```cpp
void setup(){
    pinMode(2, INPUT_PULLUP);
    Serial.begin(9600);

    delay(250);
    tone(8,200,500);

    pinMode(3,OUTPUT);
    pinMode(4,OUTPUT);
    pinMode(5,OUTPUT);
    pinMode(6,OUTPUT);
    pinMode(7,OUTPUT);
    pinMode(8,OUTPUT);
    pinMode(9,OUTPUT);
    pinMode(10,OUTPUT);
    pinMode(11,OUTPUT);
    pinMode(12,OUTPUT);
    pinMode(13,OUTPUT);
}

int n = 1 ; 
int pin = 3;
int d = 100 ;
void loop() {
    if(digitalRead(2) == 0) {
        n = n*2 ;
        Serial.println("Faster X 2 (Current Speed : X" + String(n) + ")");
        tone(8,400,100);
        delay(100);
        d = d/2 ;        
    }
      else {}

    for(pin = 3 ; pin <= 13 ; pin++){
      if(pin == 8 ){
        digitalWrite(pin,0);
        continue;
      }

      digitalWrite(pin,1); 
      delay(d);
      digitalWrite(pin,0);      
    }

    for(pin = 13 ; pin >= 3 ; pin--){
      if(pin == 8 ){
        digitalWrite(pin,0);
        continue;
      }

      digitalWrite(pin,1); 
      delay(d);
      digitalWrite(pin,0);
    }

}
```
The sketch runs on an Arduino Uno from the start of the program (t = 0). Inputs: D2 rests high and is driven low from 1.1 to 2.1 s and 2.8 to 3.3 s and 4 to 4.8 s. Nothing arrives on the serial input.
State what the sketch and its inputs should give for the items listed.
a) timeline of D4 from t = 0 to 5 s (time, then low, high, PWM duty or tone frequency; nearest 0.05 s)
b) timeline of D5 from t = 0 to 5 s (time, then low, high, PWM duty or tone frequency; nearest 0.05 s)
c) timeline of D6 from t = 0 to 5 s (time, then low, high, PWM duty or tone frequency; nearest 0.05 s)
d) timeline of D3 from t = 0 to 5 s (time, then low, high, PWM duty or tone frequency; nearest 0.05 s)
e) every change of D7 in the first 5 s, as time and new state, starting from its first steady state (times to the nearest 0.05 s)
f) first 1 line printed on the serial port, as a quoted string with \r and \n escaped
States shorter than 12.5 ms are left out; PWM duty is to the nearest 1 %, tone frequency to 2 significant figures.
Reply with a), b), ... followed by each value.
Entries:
a) 0.25 s low; 0.35 s high; 0.45 s low; 2.05 s high; 2.15 s low; 2.35 s high; 2.45 s low; 4.05 s high; 4.15 s low; 4.4 s high; 4.45 s low
b) 0.25 s low; 0.45 s high; 0.55 s low; 1.95 s high; 2.05 s low; 2.45 s high; 2.55 s low; 3.95 s high; 4.05 s low; 4.45 s high; 4.5 s low
c) 0.25 s low; 0.55 s high; 0.65 s low; 1.85 s high; 1.95 s low; 2.55 s high; 2.65 s low; 3.85 s high; 3.95 s low; 4.5 s high; 4.55 s low
d) 0.25 s high; 0.35 s low; 2.15 s high; 2.35 s low; 4.15 s high; 4.25 s low; 4.35 s high; 4.4 s low
e) 0.25 s low; 0.65 s high; 0.75 s low; 1.75 s high; 1.85 s low; 2.65 s high; 2.75 s low; 3.75 s high; 3.85 s low; 4.55 s high; 4.6 s low
f) "Faster X 2 (Current Speed : X2)\r\n"
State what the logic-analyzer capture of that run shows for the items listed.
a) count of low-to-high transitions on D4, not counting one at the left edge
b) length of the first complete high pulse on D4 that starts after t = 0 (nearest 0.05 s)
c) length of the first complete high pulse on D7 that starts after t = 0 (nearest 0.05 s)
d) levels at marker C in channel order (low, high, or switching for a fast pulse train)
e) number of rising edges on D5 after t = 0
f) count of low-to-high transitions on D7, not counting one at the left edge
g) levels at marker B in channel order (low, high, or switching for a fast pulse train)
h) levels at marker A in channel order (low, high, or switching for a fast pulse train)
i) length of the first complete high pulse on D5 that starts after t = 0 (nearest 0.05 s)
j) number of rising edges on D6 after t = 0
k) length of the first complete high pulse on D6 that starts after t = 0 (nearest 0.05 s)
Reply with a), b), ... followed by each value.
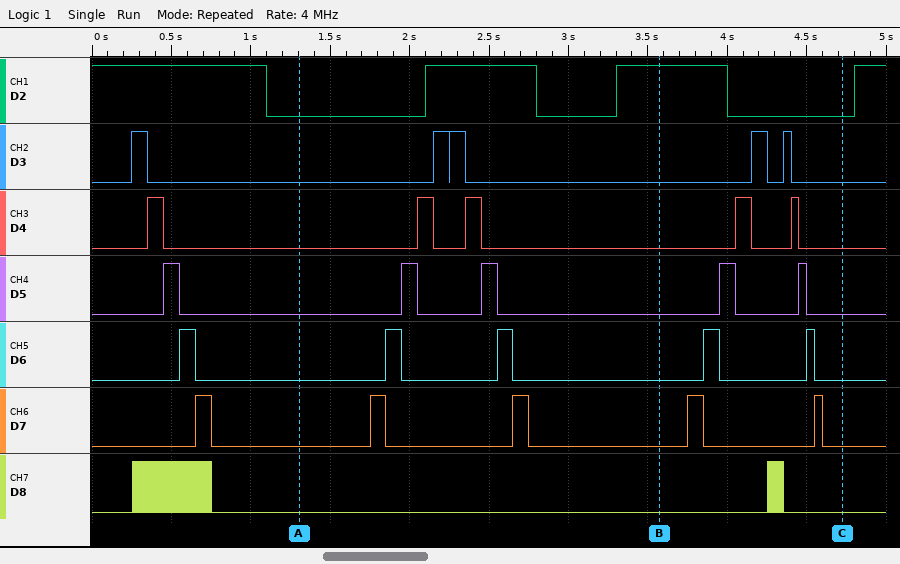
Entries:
a) 5
b) 0.10 s
c) 0.10 s
d) D2 low, D3 low, D4 low, D5 low, D6 low, D7 low, D8 low
e) 5
f) 5
g) D2 high, D3 low, D4 low, D5 low, D6 low, D7 low, D8 low
h) D2 low, D3 low, D4 low, D5 low, D6 low, D7 low, D8 low
i) 0.10 s
j) 5
k) 0.10 s
